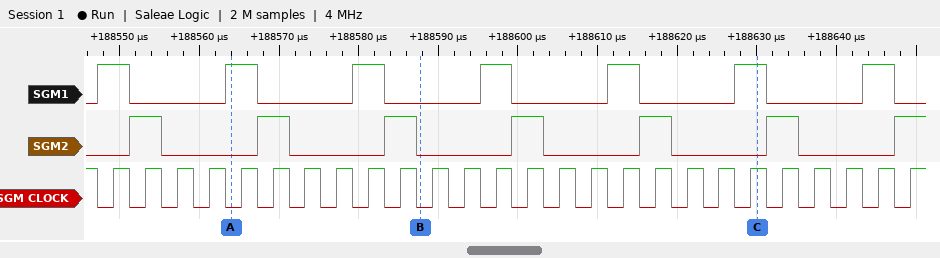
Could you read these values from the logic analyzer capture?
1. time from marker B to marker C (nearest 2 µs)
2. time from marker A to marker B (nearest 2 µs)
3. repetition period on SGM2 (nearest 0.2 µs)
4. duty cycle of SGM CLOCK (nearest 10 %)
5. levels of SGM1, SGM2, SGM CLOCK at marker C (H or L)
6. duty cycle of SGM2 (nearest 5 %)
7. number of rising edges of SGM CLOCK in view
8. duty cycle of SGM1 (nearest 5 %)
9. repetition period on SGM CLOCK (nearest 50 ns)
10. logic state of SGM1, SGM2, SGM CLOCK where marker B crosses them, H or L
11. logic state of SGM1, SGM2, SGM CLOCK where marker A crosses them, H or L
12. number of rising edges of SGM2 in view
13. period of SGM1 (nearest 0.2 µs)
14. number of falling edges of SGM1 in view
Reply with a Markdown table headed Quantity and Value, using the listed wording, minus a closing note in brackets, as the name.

| Quantity | Value |
|---|---|
| time from marker B to marker C | 42 µs |
| time from marker A to marker B | 24 µs |
| repetition period on SGM2 | 16 µs |
| duty cycle of SGM CLOCK | 50 % |
| levels of SGM1, SGM2, SGM CLOCK at marker C | SGM1=H, SGM2=L, SGM CLOCK=H |
| duty cycle of SGM2 | 25 % |
| number of rising edges of SGM CLOCK in view | 26 |
| duty cycle of SGM1 | 25 % |
| repetition period on SGM CLOCK | 4000 ns |
| logic state of SGM1, SGM2, SGM CLOCK where marker B crosses them, H or L | SGM1=L, SGM2=L, SGM CLOCK=L |
| logic state of SGM1, SGM2, SGM CLOCK where marker A crosses them, H or L | SGM1=H, SGM2=L, SGM CLOCK=L |
| number of rising edges of SGM2 in view | 7 |
| period of SGM1 | 16 µs |
| number of falling edges of SGM1 in view | 7 |
